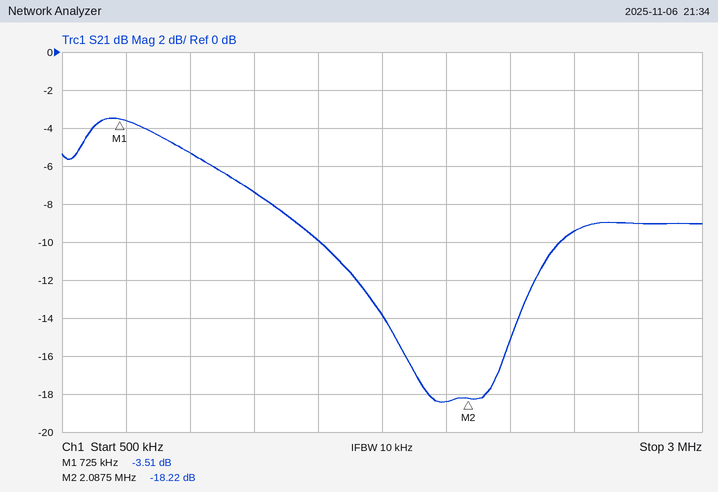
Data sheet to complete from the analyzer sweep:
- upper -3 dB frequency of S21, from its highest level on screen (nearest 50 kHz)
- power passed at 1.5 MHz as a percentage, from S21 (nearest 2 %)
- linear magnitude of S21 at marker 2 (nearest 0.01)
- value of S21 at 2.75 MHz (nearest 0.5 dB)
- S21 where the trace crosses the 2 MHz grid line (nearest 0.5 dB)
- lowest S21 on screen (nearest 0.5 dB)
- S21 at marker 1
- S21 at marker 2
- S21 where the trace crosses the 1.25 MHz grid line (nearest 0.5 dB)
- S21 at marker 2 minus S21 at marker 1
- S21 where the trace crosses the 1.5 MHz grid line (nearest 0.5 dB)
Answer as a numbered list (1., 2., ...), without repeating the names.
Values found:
1. 1.15 MHz
2. 10 %
3. 0.12
4. -9.0 dB
5. -18.5 dB
6. -18.5 dB
7. -3.51 dB
8. -18.22 dB
9. -7.5 dB
10. -14.71 dB
11. -10.0 dB
